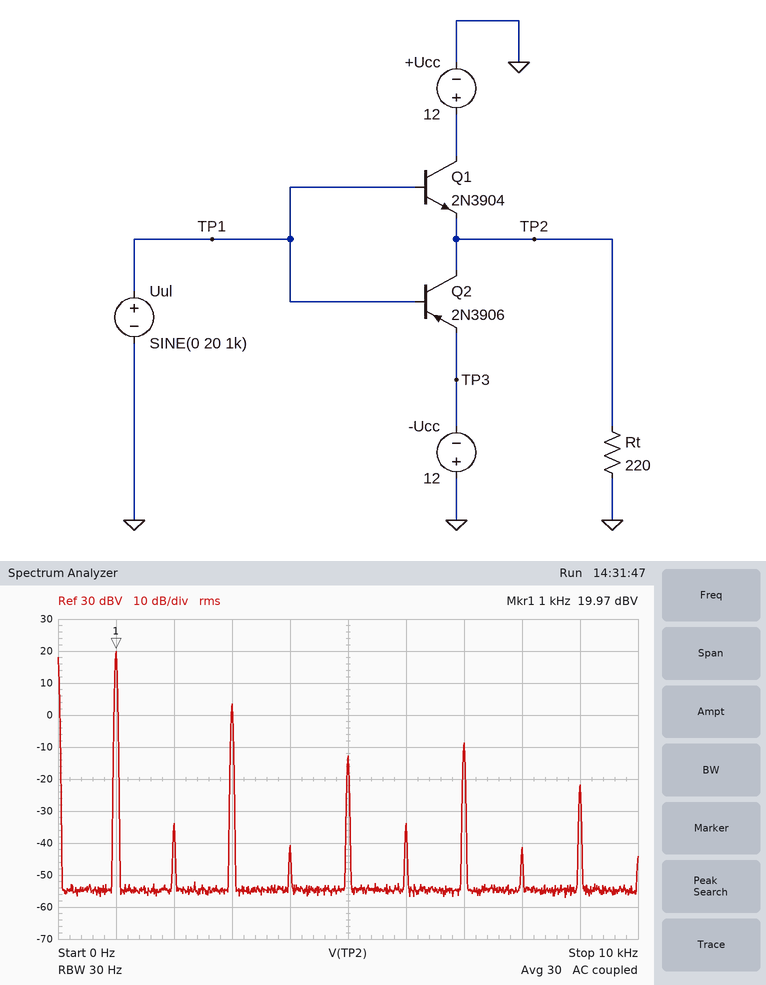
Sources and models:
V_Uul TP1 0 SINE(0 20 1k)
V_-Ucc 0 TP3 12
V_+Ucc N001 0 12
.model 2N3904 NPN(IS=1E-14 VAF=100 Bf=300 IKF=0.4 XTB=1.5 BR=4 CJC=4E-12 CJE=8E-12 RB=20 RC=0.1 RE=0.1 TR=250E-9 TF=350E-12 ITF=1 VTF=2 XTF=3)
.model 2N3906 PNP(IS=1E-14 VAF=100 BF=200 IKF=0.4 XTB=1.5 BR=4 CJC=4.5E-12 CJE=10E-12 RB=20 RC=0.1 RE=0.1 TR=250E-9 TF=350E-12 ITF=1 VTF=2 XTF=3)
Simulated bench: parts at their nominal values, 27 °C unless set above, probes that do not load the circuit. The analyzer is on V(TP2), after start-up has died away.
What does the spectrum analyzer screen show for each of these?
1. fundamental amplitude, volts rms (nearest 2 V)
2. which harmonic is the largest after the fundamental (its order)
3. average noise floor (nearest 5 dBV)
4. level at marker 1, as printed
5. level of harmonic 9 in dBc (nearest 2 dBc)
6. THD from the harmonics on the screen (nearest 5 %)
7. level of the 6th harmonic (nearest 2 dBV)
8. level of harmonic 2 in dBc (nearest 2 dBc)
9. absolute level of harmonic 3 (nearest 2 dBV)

10 V
3
-55 dBV
19.97 dBV
-42 dBc
15 %
-34 dBV
-54 dBc
4 dBV
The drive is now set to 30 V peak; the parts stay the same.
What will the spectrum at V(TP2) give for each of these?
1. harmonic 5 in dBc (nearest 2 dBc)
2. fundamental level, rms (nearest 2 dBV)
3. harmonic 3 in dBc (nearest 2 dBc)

-24 dBc
20 dBV
-12 dBc
